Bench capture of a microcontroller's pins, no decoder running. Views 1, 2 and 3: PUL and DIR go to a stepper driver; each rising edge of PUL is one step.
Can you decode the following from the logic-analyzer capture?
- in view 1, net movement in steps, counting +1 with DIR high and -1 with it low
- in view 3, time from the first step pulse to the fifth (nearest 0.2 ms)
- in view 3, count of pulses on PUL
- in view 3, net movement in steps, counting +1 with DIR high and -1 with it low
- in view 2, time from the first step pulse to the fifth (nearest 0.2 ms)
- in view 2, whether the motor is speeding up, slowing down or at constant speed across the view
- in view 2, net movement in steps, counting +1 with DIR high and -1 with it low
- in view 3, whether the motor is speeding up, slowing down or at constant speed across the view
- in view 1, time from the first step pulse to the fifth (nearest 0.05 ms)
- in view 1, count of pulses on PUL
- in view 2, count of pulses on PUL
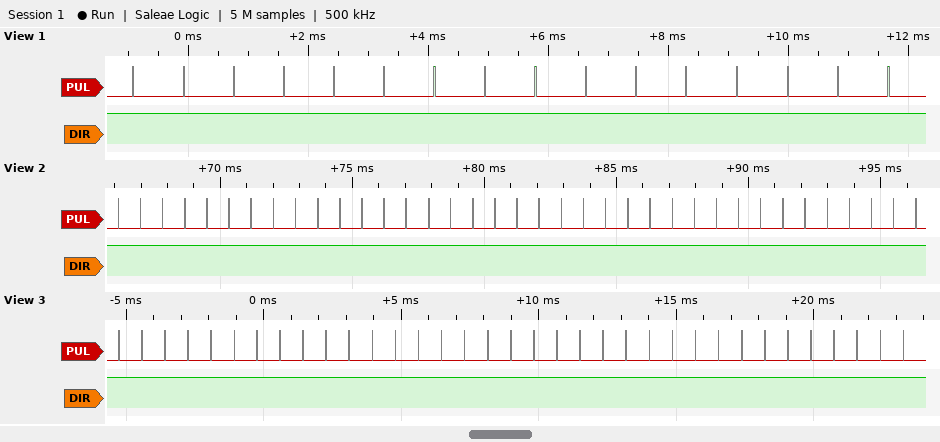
+16
3.4 ms
35
+35
3.4 ms
constant speed
+37
constant speed
3.35 ms
16
37
